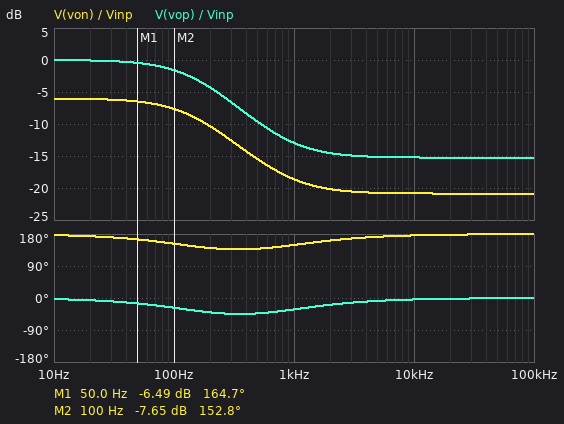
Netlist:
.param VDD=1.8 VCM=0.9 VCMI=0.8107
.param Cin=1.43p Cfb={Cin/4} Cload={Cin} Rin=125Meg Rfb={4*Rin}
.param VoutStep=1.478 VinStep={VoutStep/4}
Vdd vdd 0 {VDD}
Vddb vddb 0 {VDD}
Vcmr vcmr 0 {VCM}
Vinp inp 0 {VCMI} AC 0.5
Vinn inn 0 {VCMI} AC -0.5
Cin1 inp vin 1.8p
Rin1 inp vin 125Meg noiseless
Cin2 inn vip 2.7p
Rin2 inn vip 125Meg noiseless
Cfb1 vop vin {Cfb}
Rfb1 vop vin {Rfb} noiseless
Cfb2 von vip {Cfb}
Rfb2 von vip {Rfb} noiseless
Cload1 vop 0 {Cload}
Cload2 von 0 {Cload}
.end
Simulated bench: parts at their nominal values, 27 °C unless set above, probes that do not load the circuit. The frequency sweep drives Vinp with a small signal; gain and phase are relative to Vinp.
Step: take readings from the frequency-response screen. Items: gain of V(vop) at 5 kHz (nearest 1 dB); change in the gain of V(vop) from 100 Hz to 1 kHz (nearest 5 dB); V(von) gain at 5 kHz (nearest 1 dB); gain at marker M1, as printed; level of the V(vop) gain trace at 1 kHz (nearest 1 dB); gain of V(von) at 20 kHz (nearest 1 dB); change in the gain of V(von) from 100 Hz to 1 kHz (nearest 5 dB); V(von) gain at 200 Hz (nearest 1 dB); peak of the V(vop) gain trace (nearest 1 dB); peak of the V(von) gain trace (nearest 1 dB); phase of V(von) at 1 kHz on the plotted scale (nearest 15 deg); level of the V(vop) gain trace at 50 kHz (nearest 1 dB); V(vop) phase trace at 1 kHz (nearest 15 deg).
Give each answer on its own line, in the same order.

-15 dB
-10 dB
-21 dB
-6.49 dB
-13 dB
-21 dB
-10 dB
-10 dB
0 dB
-6 dB
150 deg
-15 dB
-30 deg
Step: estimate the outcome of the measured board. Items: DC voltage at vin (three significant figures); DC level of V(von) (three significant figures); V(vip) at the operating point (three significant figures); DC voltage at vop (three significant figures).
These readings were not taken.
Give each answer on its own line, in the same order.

811 mV
811 mV
811 mV
811 mV
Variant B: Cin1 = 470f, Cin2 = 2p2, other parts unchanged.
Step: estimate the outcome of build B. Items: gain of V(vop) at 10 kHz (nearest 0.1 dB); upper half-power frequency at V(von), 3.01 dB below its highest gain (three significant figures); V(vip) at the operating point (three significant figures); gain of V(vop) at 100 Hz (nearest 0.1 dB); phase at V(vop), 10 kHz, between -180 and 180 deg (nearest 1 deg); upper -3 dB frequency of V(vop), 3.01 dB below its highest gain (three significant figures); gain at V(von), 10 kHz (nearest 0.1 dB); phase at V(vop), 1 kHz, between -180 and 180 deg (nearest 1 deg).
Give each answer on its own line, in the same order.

-17.9 dB
151 Hz
811 mV
-1.5 dB
-8 deg
156 Hz
-21.0 dB
-40 deg
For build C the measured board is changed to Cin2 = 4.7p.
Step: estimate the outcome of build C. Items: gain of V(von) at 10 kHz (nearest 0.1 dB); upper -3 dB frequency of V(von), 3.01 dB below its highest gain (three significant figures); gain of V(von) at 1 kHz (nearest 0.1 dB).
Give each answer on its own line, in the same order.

-20.5 dB
149 Hz
-18.2 dB
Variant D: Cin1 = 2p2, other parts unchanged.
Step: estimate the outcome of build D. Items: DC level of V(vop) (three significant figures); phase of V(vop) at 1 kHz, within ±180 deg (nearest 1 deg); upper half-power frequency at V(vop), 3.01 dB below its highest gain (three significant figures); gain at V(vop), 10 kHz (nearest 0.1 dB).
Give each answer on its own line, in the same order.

811 mV
-31 deg
151 Hz
-15.0 dB
